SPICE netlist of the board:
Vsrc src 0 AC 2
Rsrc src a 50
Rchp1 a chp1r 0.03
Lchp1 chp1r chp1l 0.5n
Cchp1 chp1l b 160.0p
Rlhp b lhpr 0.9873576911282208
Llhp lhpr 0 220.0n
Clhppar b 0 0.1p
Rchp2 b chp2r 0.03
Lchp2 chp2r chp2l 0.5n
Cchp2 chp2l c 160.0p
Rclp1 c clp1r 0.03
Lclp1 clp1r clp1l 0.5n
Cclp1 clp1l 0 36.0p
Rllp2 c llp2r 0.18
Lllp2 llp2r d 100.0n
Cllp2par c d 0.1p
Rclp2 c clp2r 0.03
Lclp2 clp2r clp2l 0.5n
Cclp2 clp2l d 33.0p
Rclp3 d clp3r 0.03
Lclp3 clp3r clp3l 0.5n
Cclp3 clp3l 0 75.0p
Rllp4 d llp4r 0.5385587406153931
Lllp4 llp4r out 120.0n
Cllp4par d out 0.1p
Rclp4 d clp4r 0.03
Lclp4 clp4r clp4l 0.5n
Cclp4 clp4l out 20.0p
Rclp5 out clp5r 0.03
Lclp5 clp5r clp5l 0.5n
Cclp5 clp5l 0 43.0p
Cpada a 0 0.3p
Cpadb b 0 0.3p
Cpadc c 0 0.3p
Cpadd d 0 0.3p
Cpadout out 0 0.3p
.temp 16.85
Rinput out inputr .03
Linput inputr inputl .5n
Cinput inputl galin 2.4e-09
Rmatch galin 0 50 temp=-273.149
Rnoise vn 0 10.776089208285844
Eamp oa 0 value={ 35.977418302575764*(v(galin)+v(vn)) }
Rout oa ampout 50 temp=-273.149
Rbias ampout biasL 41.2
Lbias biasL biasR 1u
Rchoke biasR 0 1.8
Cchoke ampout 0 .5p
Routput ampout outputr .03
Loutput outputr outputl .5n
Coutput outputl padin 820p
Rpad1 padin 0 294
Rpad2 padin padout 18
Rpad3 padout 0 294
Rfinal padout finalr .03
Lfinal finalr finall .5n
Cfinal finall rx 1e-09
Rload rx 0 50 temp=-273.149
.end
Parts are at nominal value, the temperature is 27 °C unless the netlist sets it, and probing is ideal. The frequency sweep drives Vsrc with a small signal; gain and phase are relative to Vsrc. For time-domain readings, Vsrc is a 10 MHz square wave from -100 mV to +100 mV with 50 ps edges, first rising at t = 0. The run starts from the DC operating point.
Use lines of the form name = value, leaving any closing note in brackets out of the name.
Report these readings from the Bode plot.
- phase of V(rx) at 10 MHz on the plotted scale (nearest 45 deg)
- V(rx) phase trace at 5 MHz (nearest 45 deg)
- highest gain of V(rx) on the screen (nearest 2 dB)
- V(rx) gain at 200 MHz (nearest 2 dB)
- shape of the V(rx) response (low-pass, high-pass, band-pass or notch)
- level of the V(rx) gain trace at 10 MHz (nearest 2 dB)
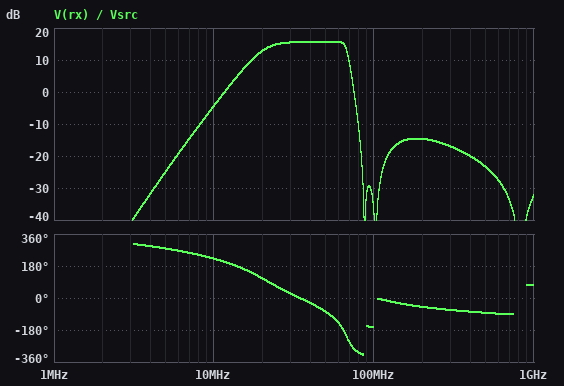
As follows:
phase of V(rx) at 10 MHz on the plotted scale = 225 deg
V(rx) phase trace at 5 MHz = 270 deg
highest gain of V(rx) on the screen = 16 dB
V(rx) gain at 200 MHz = -14 dB
shape of the V(rx) response = band-pass
level of the V(rx) gain trace at 10 MHz = -4 dB
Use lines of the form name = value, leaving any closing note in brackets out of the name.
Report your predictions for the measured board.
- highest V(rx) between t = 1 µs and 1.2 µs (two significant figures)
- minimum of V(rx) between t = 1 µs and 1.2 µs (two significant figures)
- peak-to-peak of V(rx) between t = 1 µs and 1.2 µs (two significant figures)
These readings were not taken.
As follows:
highest V(rx) between t = 1 µs and 1.2 µs = 500 mV
minimum of V(rx) between t = 1 µs and 1.2 µs = -500 mV
peak-to-peak of V(rx) between t = 1 µs and 1.2 µs = 1.0 V
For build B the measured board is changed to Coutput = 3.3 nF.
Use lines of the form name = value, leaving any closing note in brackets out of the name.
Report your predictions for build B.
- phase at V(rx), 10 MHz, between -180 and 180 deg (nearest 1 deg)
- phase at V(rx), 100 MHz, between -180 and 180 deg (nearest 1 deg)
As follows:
phase at V(rx), 10 MHz, between -180 and 180 deg = -149 deg
phase at V(rx), 100 MHz, between -180 and 180 deg = -164 deg
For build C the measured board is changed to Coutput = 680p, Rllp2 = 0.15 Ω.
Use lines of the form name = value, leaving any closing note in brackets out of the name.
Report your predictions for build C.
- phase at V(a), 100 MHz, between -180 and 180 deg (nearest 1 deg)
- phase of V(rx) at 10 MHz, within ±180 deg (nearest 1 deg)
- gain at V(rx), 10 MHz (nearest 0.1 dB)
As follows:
phase at V(a), 100 MHz, between -180 and 180 deg = -33 deg
phase of V(rx) at 10 MHz, within ±180 deg = -136 deg
gain at V(rx), 10 MHz = -4.4 dB
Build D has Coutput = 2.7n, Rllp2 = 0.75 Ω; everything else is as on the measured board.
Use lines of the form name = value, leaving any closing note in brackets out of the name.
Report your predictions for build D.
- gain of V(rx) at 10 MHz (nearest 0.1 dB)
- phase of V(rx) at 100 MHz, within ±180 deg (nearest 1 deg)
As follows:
gain of V(rx) at 10 MHz = -4.2 dB
phase of V(rx) at 100 MHz, within ±180 deg = -165 deg
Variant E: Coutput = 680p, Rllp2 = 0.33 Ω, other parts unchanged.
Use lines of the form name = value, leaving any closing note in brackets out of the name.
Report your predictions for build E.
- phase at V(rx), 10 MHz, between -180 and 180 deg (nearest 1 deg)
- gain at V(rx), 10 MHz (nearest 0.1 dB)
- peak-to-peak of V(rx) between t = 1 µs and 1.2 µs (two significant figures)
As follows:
phase at V(rx), 10 MHz, between -180 and 180 deg = -136 deg
gain at V(rx), 10 MHz = -4.4 dB
peak-to-peak of V(rx) between t = 1 µs and 1.2 µs = 1.0 V
